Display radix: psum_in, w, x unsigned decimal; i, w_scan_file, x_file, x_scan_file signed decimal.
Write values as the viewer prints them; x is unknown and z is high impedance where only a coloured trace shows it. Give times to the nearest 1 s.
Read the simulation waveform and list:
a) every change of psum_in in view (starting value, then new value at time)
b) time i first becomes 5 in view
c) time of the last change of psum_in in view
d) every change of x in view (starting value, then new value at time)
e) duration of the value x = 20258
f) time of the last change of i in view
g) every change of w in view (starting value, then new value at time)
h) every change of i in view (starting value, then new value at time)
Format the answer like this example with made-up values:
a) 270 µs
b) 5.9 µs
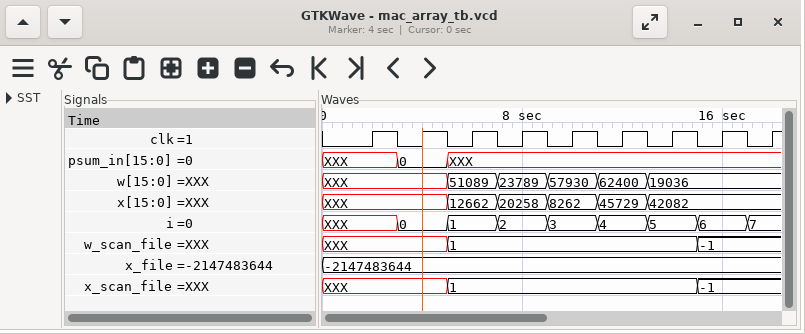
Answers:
a) XXX, 0 at 3 s, XXX at 5 s
b) 13 s
c) 5 s
d) XXX, 12662 at 5 s, 20258 at 7 s, 8262 at 9 s, 45729 at 11 s, 42082 at 13 s
e) 2 s
f) 17 s
g) XXX, 51089 at 5 s, 23789 at 7 s, 57930 at 9 s, 62400 at 11 s, 19036 at 13 s
h) XXX, 0 at 3 s, 1 at 5 s, 2 at 7 s, 3 at 9 s, 4 at 11 s, 5 at 13 s, 6 at 15 s, 7 at 17 s
